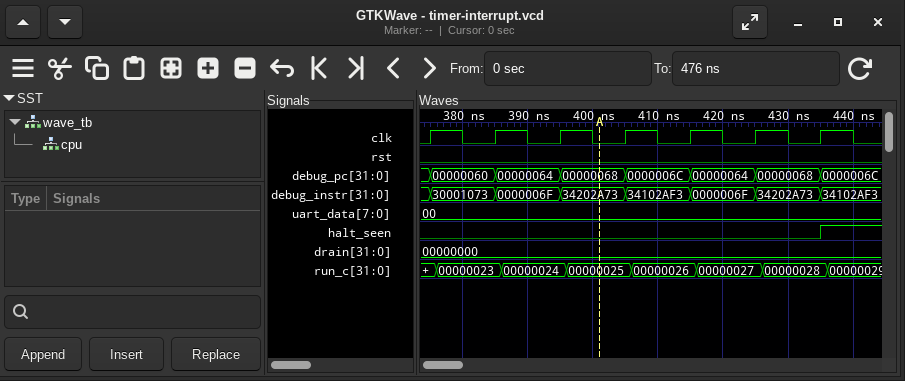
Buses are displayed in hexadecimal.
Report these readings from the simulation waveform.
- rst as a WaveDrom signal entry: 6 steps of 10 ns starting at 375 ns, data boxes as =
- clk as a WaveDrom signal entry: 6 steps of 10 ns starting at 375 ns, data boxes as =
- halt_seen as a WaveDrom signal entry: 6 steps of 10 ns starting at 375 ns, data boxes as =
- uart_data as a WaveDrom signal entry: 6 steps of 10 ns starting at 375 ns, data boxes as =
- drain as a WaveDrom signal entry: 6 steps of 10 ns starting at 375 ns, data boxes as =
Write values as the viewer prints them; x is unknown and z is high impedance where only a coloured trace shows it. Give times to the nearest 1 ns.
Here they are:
{name: 'rst', wave: '0.....'}
{name: 'clk', wave: 'p.....'}
{name: 'halt_seen', wave: '0.....'}
{name: 'uart_data', wave: '=.....', data: '00'}
{name: 'drain', wave: '=.....', data: '00000000'}
